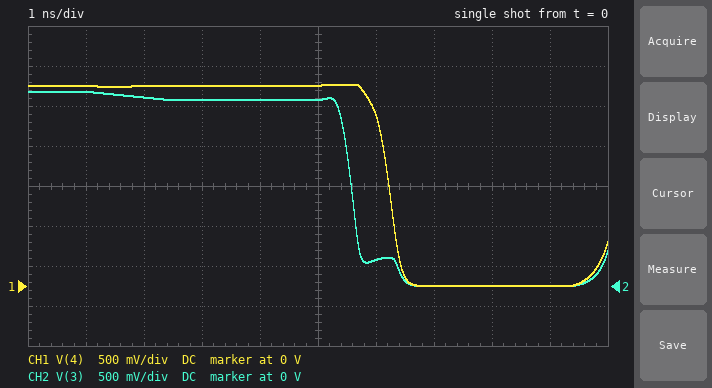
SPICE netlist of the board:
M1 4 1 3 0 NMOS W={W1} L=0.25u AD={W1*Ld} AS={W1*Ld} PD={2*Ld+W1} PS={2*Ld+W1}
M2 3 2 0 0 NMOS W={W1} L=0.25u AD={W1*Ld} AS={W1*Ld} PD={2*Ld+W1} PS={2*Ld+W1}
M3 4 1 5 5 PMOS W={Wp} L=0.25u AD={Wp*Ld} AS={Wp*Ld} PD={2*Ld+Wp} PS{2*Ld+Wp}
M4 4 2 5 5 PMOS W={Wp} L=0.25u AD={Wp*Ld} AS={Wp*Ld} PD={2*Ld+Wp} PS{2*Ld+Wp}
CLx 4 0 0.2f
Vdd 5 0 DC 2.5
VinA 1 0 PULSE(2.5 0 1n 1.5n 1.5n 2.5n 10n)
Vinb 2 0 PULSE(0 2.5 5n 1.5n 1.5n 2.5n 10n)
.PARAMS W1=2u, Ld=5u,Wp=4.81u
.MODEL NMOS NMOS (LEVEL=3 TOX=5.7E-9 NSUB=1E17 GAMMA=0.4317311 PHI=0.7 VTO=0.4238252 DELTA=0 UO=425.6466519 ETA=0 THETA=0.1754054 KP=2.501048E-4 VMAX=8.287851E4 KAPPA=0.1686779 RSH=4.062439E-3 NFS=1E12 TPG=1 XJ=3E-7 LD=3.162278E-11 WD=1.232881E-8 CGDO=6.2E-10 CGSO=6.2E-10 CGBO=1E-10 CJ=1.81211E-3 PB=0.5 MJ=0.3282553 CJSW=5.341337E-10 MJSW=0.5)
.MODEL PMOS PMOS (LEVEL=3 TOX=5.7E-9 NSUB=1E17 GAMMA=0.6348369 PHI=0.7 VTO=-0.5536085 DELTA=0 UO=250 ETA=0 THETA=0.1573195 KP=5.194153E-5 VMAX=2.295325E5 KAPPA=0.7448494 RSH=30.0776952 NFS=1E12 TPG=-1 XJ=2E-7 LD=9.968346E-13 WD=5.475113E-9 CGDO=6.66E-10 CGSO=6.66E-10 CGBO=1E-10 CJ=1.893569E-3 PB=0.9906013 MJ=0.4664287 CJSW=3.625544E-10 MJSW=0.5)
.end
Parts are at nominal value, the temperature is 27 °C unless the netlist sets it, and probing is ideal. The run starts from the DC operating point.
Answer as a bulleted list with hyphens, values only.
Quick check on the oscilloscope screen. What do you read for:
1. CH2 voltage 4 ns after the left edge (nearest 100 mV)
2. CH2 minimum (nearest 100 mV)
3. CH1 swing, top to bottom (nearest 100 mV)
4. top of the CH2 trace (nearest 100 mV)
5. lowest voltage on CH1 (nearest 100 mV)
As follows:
- 2.3 V
- 0 V
- 2.5 V
- 2.4 V
- 0 V
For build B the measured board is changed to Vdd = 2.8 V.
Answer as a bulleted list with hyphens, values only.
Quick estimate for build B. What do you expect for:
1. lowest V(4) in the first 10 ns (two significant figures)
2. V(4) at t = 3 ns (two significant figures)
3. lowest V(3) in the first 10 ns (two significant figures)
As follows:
- -3.2 mV
- 2.8 V
- -2.4 mV
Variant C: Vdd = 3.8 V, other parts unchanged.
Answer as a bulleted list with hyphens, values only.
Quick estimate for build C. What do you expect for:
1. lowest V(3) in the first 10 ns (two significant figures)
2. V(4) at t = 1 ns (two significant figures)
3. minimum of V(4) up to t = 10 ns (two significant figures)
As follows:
- 300 mV
- 3.8 V
- 690 mV
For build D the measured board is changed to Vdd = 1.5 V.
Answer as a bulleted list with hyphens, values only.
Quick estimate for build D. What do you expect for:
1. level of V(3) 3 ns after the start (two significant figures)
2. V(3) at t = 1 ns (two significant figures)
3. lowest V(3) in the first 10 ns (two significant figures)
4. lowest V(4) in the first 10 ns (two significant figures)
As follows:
- 1.4 V
- 1.5 V
- -6.3 mV
- -7.6 mV
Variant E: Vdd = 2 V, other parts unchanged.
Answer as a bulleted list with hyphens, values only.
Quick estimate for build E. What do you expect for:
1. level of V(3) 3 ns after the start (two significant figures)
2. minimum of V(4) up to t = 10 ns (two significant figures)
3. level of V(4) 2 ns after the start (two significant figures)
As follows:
- 1.9 V
- -5.9 mV
- 2.0 V
